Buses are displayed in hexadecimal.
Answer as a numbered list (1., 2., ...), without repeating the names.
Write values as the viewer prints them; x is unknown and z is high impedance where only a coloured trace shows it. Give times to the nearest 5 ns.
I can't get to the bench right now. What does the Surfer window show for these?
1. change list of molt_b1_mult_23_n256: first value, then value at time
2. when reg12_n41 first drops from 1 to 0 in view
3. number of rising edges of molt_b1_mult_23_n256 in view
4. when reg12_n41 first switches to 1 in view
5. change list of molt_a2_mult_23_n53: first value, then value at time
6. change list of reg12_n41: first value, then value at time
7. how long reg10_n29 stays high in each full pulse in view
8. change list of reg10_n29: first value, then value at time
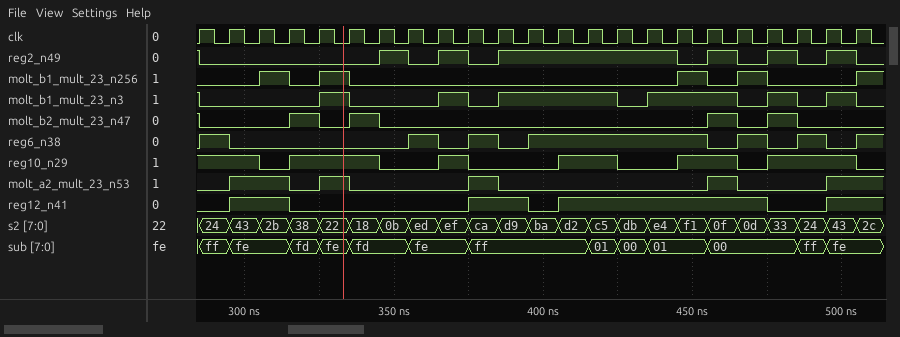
1. 0, 1 at 305 ns, 0 at 315 ns, 1 at 325 ns, 0 at 335 ns, 1 at 445 ns, 0 at 455 ns, 1 at 465 ns, 0 at 475 ns, 1 at 505 ns
2. 315 ns
3. 5
4. 295 ns
5. 0, 1 at 295 ns, 0 at 315 ns, 1 at 325 ns, 0 at 335 ns, 1 at 375 ns, 0 at 385 ns, 1 at 455 ns, 0 at 465 ns, 1 at 495 ns
6. 0, 1 at 295 ns, 0 at 315 ns, 1 at 375 ns, 0 at 395 ns, 1 at 405 ns, 0 at 475 ns, 1 at 495 ns
7. 30 ns, 10 ns, 20 ns, 20 ns, 30 ns
8. 1, 0 at 305 ns, 1 at 315 ns, 0 at 345 ns, 1 at 365 ns, 0 at 375 ns, 1 at 405 ns, 0 at 425 ns, 1 at 445 ns, 0 at 465 ns, 1 at 475 ns, 0 at 505 ns
